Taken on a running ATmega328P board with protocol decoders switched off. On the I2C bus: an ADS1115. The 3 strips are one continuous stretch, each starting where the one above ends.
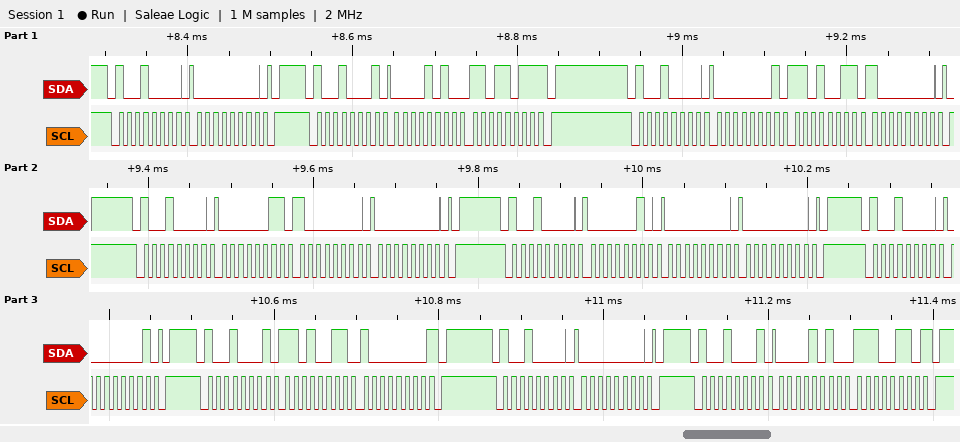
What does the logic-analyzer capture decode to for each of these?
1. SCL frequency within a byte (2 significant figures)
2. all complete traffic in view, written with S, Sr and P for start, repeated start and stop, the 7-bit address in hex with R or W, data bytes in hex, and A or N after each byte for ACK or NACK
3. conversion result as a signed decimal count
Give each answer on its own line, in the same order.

100 kHz
S 48W A 00 A P S 48R A 0A A DB N P S 48W A 01 A D3 A 80 A P S 48W A 03 A 80 A 00 A P S 48W A 02 A 00 A 00 A P S 48W A 01 A P S 48R A D3 A 80 N P S 48W A 00 A P S 48R A 0A A E6 N P
2779
